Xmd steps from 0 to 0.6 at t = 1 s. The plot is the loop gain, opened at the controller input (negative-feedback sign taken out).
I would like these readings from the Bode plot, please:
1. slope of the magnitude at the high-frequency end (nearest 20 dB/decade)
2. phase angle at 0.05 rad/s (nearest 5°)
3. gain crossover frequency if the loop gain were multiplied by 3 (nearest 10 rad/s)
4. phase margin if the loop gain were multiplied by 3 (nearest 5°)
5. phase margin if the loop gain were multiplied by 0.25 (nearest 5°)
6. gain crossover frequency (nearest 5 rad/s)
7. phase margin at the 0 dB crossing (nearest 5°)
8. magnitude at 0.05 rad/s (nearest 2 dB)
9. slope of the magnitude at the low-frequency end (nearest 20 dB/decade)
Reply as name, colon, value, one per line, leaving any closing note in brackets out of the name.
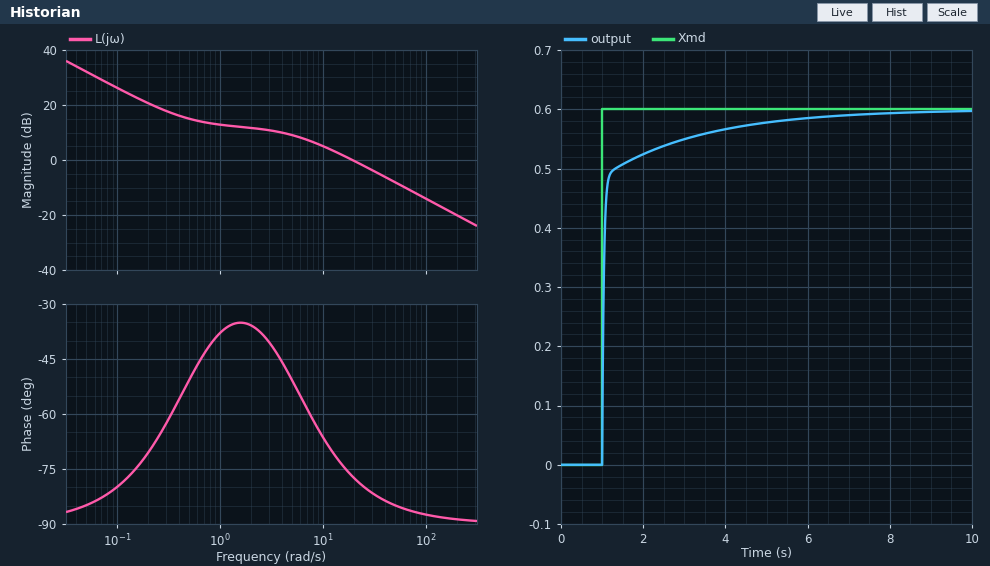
slope of the magnitude at the high-frequency end: -20 dB/decade
phase angle at 0.05 rad/s: -85°
gain crossover frequency if the loop gain were multiplied by 3: 60 rad/s
phase margin if the loop gain were multiplied by 3: 95°
phase margin if the loop gain were multiplied by 0.25: 145°
gain crossover frequency: 20 rad/s
phase margin at the 0 dB crossing: 105°
magnitude at 0.05 rad/s: 32 dB
slope of the magnitude at the low-frequency end: -20 dB/decade
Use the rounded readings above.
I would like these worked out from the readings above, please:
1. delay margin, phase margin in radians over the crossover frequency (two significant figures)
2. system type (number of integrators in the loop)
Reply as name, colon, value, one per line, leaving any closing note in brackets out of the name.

delay margin, phase margin in radians over the crossover frequency: 0.092 s
system type: 1
